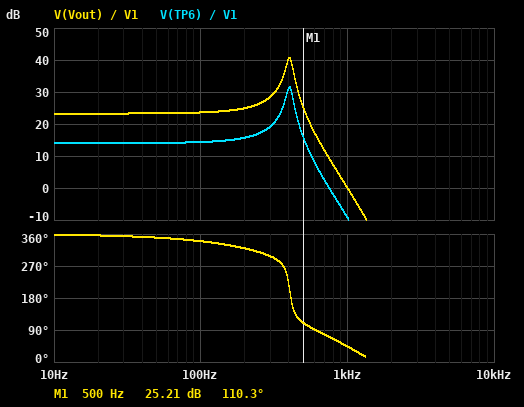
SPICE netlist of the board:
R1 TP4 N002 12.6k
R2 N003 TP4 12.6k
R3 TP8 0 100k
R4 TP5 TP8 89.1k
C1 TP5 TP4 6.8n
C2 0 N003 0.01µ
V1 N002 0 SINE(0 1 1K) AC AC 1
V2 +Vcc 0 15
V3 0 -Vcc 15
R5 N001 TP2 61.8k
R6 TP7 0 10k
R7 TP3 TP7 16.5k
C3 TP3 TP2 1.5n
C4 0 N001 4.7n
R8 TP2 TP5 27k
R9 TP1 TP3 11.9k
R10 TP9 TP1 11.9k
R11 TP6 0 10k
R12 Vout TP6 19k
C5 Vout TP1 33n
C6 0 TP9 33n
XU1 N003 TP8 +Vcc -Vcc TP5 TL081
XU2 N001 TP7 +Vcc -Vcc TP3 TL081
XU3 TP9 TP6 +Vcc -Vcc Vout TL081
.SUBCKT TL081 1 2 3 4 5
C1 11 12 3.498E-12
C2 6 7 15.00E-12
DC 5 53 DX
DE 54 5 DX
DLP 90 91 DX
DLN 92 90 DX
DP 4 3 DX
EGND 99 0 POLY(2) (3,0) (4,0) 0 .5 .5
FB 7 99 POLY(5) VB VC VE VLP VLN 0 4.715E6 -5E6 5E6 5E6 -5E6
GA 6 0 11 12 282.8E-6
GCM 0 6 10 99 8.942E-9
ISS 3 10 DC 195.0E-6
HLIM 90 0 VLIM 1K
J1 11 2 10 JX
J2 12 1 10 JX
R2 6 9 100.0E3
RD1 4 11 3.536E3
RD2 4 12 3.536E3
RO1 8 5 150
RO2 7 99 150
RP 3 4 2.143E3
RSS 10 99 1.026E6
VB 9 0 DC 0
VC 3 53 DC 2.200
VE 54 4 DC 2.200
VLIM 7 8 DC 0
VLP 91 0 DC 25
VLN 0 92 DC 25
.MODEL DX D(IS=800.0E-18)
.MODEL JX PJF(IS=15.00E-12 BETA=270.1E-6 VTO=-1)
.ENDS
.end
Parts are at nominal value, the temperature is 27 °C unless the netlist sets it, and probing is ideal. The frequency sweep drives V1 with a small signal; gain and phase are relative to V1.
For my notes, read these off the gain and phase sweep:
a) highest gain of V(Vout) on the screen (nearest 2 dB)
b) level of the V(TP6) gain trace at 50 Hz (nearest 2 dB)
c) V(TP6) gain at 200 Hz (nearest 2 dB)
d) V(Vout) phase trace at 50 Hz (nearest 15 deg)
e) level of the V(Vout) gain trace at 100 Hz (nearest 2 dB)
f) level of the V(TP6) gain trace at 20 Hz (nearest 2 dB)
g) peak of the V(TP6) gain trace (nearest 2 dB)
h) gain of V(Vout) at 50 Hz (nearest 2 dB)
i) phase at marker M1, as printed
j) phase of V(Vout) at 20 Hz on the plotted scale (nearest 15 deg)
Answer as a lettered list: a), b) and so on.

a) 40 dB
b) 14 dB
c) 16 dB
d) 345 deg
e) 24 dB
f) 14 dB
g) 32 dB
h) 24 dB
i) 110.3 deg
j) 360 deg
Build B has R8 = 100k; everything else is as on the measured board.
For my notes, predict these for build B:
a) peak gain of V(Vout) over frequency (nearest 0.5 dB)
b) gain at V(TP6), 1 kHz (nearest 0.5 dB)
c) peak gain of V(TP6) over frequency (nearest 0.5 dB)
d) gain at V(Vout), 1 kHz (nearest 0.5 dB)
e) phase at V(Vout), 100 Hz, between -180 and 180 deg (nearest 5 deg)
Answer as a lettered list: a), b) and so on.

a) 39.5 dB
b) -12.5 dB
c) 30.5 dB
d) -3.0 dB
e) -25 deg
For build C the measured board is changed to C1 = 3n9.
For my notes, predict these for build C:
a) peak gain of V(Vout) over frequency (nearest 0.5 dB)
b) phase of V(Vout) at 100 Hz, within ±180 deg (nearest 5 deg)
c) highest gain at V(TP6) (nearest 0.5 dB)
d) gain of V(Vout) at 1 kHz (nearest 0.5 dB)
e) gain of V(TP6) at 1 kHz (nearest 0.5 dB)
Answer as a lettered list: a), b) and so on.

a) 40.5 dB
b) -20 deg
c) 31.0 dB
d) -1.5 dB
e) -11.0 dB
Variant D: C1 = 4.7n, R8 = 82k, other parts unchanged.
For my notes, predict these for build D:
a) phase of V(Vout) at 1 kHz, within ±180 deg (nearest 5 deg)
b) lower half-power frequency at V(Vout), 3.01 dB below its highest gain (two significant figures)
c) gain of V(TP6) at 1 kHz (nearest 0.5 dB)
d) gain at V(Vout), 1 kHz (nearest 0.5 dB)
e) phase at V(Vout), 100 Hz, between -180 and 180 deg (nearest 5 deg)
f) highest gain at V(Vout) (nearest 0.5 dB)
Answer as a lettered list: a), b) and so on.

a) 25 deg
b) 380 Hz
c) -13.0 dB
d) -3.5 dB
e) -25 deg
f) 39.5 dB
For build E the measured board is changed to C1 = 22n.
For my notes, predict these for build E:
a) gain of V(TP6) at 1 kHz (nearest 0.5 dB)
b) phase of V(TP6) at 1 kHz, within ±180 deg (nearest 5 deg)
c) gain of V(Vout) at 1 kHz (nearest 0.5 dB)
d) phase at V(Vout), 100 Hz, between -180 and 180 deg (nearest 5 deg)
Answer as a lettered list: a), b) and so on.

a) 1.0 dB
b) -70 deg
c) 10.5 dB
d) -15 deg
